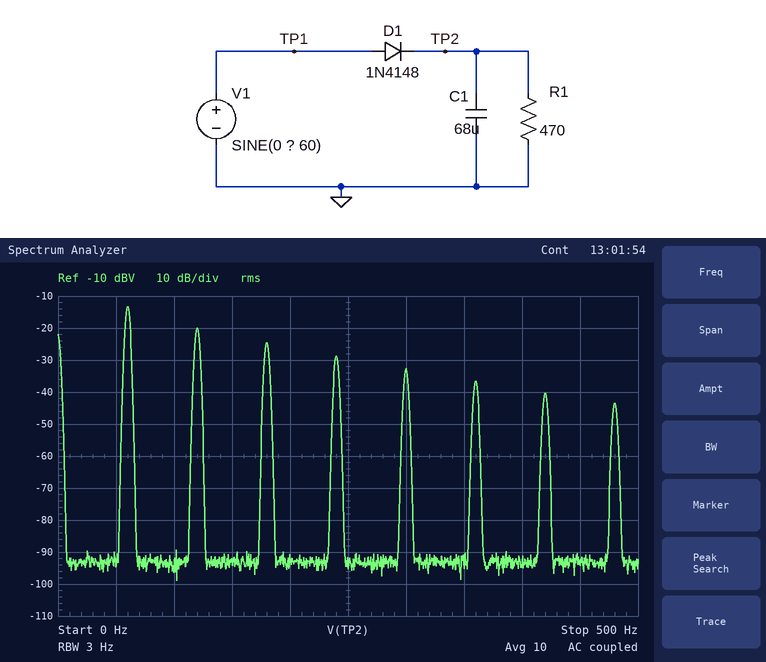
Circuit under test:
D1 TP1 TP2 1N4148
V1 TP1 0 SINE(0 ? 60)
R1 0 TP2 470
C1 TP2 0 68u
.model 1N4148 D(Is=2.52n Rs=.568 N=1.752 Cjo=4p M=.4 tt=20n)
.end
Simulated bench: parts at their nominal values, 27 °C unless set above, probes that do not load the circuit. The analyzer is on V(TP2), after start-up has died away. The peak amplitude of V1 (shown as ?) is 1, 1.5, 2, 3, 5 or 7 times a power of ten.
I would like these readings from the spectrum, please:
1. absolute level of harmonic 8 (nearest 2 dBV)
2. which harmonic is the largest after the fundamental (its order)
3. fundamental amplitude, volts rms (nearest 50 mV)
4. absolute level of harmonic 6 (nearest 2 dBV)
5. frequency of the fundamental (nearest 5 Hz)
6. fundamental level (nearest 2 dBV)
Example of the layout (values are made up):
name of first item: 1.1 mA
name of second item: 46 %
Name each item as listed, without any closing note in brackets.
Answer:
absolute level of harmonic 8: -44 dBV
which harmonic is the largest after the fundamental: 2
fundamental amplitude, volts rms: 200 mV
absolute level of harmonic 6: -36 dBV
frequency of the fundamental: 60 Hz
fundamental level: -14 dBV
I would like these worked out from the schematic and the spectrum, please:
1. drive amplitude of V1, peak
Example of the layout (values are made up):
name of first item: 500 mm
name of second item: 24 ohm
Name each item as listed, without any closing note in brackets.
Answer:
drive amplitude of V1, peak: 3 V
